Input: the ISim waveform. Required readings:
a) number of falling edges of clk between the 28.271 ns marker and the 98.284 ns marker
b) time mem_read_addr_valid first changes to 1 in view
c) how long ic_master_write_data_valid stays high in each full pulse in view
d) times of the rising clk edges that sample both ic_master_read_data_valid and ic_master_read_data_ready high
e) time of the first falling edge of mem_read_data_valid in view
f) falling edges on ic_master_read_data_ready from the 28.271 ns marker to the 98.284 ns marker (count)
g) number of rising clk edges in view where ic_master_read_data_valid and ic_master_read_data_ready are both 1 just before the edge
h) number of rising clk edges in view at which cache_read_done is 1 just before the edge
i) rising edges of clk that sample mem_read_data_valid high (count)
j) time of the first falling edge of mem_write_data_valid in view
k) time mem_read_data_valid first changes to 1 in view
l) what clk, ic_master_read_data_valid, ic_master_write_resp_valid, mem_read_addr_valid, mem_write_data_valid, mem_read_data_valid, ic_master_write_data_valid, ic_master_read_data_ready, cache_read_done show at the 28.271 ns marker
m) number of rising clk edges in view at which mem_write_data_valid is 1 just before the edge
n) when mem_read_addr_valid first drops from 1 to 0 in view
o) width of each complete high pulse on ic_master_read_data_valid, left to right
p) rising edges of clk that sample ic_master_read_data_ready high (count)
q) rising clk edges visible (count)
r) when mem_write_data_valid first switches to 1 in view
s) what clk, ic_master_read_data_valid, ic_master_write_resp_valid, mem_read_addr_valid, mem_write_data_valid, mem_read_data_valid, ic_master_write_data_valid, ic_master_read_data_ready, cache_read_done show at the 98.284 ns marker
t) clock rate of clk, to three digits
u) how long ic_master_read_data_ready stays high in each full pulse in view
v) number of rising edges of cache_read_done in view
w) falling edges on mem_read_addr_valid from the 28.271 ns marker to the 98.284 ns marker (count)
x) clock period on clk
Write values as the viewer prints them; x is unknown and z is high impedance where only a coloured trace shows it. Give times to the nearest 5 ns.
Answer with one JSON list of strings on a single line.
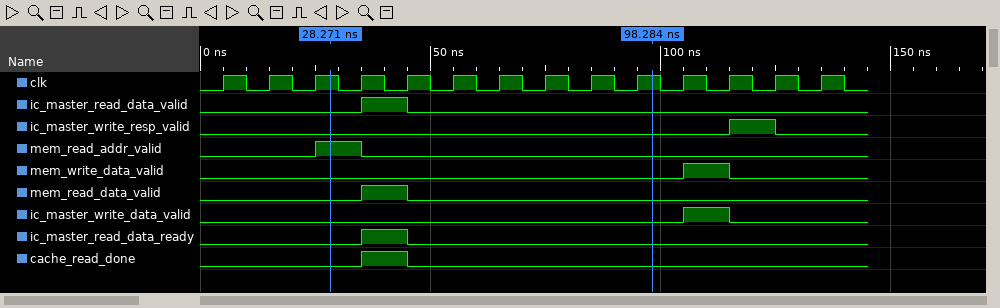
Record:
["7", "25 ns", "10 ns", "45 ns", "45 ns", "1", "1", "1", "1", "115 ns", "35 ns", "clk=1, ic_master_read_data_valid=0, ic_master_write_resp_valid=0, mem_read_addr_valid=1, mem_write_data_valid=0, mem_read_data_valid=0, ic_master_write_data_valid=0, ic_master_read_data_ready=0, cache_read_done=0", "1", "35 ns", "10 ns", "1", "14", "105 ns", "clk=1, ic_master_read_data_valid=0, ic_master_write_resp_valid=0, mem_read_addr_valid=0, mem_write_data_valid=0, mem_read_data_valid=0, ic_master_write_data_valid=0, ic_master_read_data_ready=0, cache_read_done=0", "100 MHz", "10 ns", "1", "1", "10 ns"]
